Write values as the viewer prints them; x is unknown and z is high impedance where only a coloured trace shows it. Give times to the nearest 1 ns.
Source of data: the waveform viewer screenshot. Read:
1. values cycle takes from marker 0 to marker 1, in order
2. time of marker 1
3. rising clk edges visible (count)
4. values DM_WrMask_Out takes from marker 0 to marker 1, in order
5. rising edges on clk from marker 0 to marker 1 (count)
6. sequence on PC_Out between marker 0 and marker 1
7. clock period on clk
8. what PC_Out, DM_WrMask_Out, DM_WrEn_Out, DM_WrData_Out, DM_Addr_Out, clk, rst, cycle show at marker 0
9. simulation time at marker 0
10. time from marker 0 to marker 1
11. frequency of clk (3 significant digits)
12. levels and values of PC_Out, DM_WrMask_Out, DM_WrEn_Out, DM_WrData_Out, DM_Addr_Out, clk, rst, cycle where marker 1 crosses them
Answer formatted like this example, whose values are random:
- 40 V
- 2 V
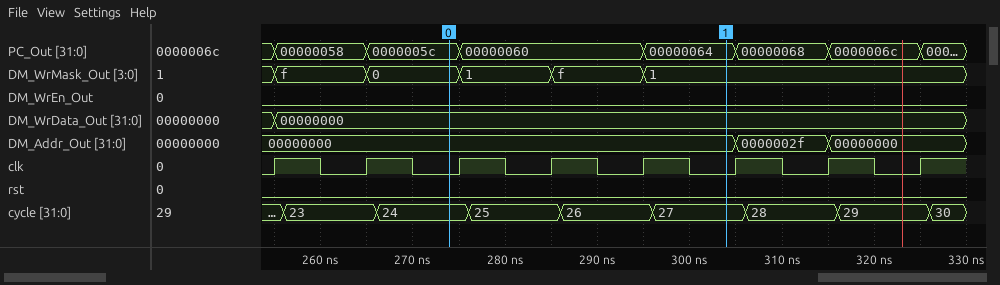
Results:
- 24, 25, 26, 27
- 304 ns
- 8
- 0, 1, f, 1
- 3
- 0000005c, 00000060, 00000064
- 10 ns
- PC_Out=0000005c, DM_WrMask_Out=0, DM_WrEn_Out=0, DM_WrData_Out=00000000, DM_Addr_Out=00000000, clk=0, rst=0, cycle=24
- 274 ns
- 30 ns
- 100 MHz
- PC_Out=00000064, DM_WrMask_Out=1, DM_WrEn_Out=0, DM_WrData_Out=00000000, DM_Addr_Out=00000000, clk=0, rst=0, cycle=27
